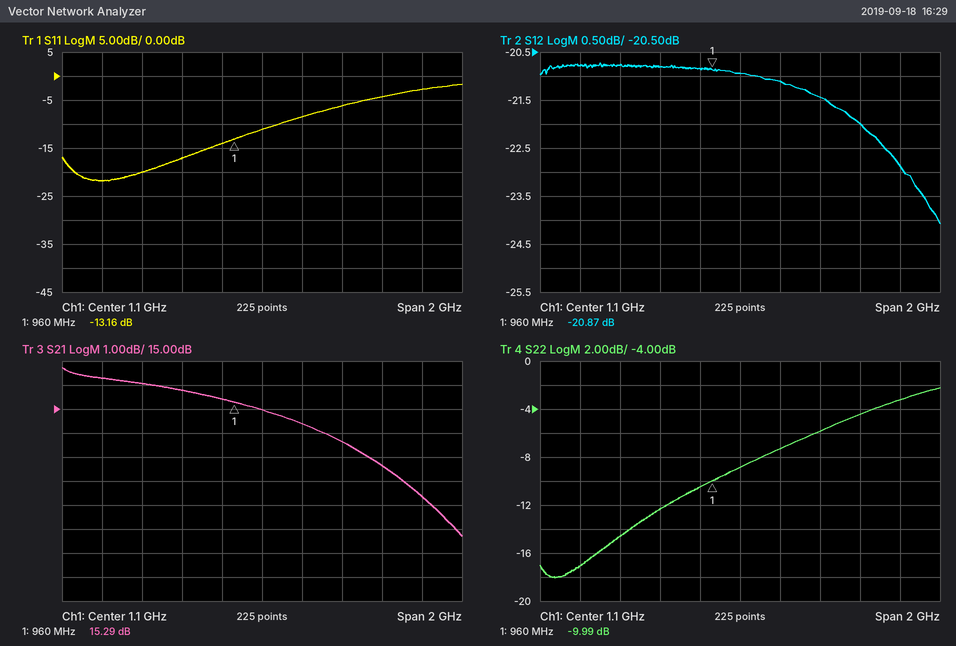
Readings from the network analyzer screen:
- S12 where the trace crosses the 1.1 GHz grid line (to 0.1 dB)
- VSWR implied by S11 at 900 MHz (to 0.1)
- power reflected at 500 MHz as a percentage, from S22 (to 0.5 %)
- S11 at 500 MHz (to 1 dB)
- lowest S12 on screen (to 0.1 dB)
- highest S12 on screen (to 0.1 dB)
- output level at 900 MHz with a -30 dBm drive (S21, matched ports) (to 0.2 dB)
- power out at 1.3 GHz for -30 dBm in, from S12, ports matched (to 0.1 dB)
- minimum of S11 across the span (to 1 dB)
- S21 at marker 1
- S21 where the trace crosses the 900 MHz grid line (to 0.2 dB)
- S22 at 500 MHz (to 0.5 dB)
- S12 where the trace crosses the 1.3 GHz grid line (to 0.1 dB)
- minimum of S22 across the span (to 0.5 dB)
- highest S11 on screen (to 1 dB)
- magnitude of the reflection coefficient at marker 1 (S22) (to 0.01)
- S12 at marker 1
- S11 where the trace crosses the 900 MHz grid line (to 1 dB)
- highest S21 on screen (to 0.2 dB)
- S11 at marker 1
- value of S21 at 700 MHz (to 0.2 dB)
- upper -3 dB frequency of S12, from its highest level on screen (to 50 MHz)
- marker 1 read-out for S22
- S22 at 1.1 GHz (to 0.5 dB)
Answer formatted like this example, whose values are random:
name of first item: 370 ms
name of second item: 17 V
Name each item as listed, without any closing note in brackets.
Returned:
S12 where the trace crosses the 1.1 GHz grid line: -20.9 dB
VSWR implied by S11 at 900 MHz: 1.5
power reflected at 500 MHz as a percentage, from S22: 3.5 %
S11 at 500 MHz: -20 dB
lowest S12 on screen: -24.1 dB
highest S12 on screen: -20.7 dB
output level at 900 MHz with a -30 dBm drive (S21, matched ports): -14.6 dBm
power out at 1.3 GHz for -30 dBm in, from S12, ports matched: -51.1 dBm
minimum of S11 across the span: -22 dB
S21 at marker 1: 15.29 dB
S21 where the trace crosses the 900 MHz grid line: 15.4 dB
S22 at 500 MHz: -14.5 dB
S12 where the trace crosses the 1.3 GHz grid line: -21.1 dB
minimum of S22 across the span: -18.0 dB
highest S11 on screen: -2 dB
magnitude of the reflection coefficient at marker 1 (S22): 0.32
S12 at marker 1: -20.87 dB
S11 where the trace crosses the 900 MHz grid line: -14 dB
highest S21 on screen: 16.8 dB
S11 at marker 1: -13.16 dB
value of S21 at 700 MHz: 15.8 dB
upper -3 dB frequency of S12, from its highest level on screen: 2.05 GHz
marker 1 read-out for S22: -9.99 dB
S22 at 1.1 GHz: -9.0 dB
